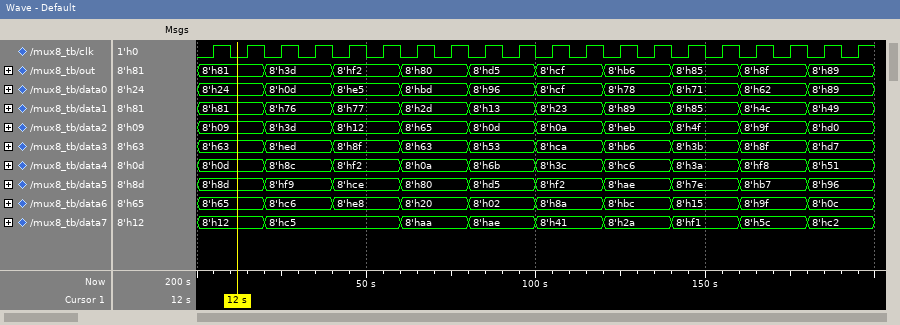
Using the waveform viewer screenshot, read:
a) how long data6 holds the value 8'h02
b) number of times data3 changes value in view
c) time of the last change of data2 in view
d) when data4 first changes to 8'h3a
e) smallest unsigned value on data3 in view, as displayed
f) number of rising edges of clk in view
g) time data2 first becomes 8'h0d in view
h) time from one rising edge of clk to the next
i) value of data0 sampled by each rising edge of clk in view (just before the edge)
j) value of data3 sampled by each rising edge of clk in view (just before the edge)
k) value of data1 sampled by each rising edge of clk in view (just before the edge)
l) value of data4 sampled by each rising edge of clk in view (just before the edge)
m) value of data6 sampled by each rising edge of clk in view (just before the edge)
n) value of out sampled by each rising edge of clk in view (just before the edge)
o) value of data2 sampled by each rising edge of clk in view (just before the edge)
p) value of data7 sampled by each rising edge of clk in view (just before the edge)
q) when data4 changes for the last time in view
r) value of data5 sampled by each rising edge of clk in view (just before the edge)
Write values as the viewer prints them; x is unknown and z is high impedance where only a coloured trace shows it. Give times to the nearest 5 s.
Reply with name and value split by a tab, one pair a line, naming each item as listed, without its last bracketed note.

how long data6 holds the value 8'h02	20 s
number of times data3 changes value in view	9
time of the last change of data2 in view	180 s
when data4 first changes to 8'h3a	140 s
smallest unsigned value on data3 in view, as displayed	8'h3b
number of rising edges of clk in view	20
time data2 first becomes 8'h0d in view	80 s
time from one rising edge of clk to the next	10 s
value of data0 sampled by each rising edge of clk in view	8'h24, 8'h24, 8'h0d, 8'h0d, 8'he5, 8'he5, 8'hbd, 8'hbd, 8'h96, 8'h96, 8'hcf, 8'hcf, 8'h78, 8'h78, 8'h71, 8'h71, 8'h62, 8'h62, 8'h89, 8'h89
value of data3 sampled by each rising edge of clk in view	8'h63, 8'h63, 8'hed, 8'hed, 8'h8f, 8'h8f, 8'h63, 8'h63, 8'h53, 8'h53, 8'hca, 8'hca, 8'hb6, 8'hb6, 8'h3b, 8'h3b, 8'h8f, 8'h8f, 8'hd7, 8'hd7
value of data1 sampled by each rising edge of clk in view	8'h81, 8'h81, 8'h76, 8'h76, 8'h77, 8'h77, 8'h2d, 8'h2d, 8'h13, 8'h13, 8'h23, 8'h23, 8'h89, 8'h89, 8'h85, 8'h85, 8'h4c, 8'h4c, 8'h49, 8'h49
value of data4 sampled by each rising edge of clk in view	8'h0d, 8'h0d, 8'h8c, 8'h8c, 8'hf2, 8'hf2, 8'h0a, 8'h0a, 8'h6b, 8'h6b, 8'h3c, 8'h3c, 8'hc6, 8'hc6, 8'h3a, 8'h3a, 8'hf8, 8'hf8, 8'h51, 8'h51
value of data6 sampled by each rising edge of clk in view	8'h65, 8'h65, 8'hc6, 8'hc6, 8'he8, 8'he8, 8'h20, 8'h20, 8'h02, 8'h02, 8'h8a, 8'h8a, 8'hbc, 8'hbc, 8'h15, 8'h15, 8'h9f, 8'h9f, 8'h0c, 8'h0c
value of out sampled by each rising edge of clk in view	8'h81, 8'h81, 8'h3d, 8'h3d, 8'hf2, 8'hf2, 8'h80, 8'h80, 8'hd5, 8'hd5, 8'hcf, 8'hcf, 8'hb6, 8'hb6, 8'h85, 8'h85, 8'h8f, 8'h8f, 8'h89, 8'h89
value of data2 sampled by each rising edge of clk in view	8'h09, 8'h09, 8'h3d, 8'h3d, 8'h12, 8'h12, 8'h65, 8'h65, 8'h0d, 8'h0d, 8'h0a, 8'h0a, 8'heb, 8'heb, 8'h4f, 8'h4f, 8'h9f, 8'h9f, 8'hd0, 8'hd0
value of data7 sampled by each rising edge of clk in view	8'h12, 8'h12, 8'hc5, 8'hc5, 8'hc5, 8'hc5, 8'haa, 8'haa, 8'hae, 8'hae, 8'h41, 8'h41, 8'h2a, 8'h2a, 8'hf1, 8'hf1, 8'h5c, 8'h5c, 8'hc2, 8'hc2
when data4 changes for the last time in view	180 s
value of data5 sampled by each rising edge of clk in view	8'h8d, 8'h8d, 8'hf9, 8'hf9, 8'hce, 8'hce, 8'h80, 8'h80, 8'hd5, 8'hd5, 8'hf2, 8'hf2, 8'hae, 8'hae, 8'h7e, 8'h7e, 8'hb7, 8'hb7, 8'h96, 8'h96
